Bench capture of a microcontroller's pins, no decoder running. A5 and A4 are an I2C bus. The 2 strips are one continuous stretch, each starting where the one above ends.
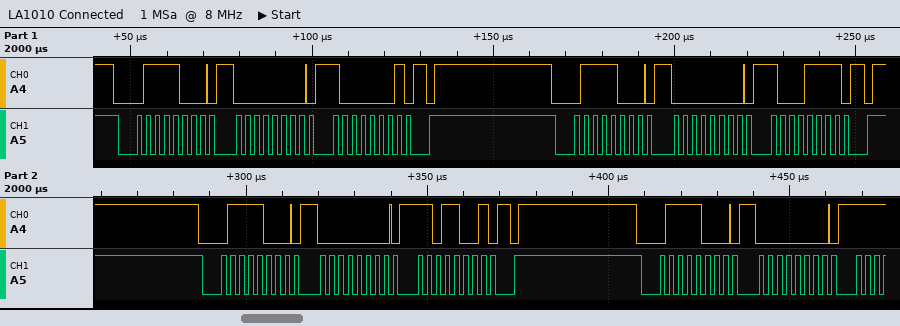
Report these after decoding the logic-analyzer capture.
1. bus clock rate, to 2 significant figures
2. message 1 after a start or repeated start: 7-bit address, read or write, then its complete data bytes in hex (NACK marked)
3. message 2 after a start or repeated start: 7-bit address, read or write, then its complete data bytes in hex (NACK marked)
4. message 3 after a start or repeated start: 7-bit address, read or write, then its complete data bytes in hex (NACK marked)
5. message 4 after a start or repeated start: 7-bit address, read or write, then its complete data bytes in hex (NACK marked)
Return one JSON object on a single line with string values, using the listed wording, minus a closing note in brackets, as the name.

{"bus clock rate, to 2 significant figures": "400 kHz", "message 1 after a start or repeated start: 7-bit address, read or write, then its complete data bytes in hex": "0x3C write: 00 81", "message 2 after a start or repeated start: 7-bit address, read or write, then its complete data bytes in hex": "0x3C write: 00 8F", "message 3 after a start or repeated start: 7-bit address, read or write, then its complete data bytes in hex": "0x3C write: 00 D9", "message 4 after a start or repeated start: 7-bit address, read or write, then its complete data bytes in hex": "0x3C write: 00"}
